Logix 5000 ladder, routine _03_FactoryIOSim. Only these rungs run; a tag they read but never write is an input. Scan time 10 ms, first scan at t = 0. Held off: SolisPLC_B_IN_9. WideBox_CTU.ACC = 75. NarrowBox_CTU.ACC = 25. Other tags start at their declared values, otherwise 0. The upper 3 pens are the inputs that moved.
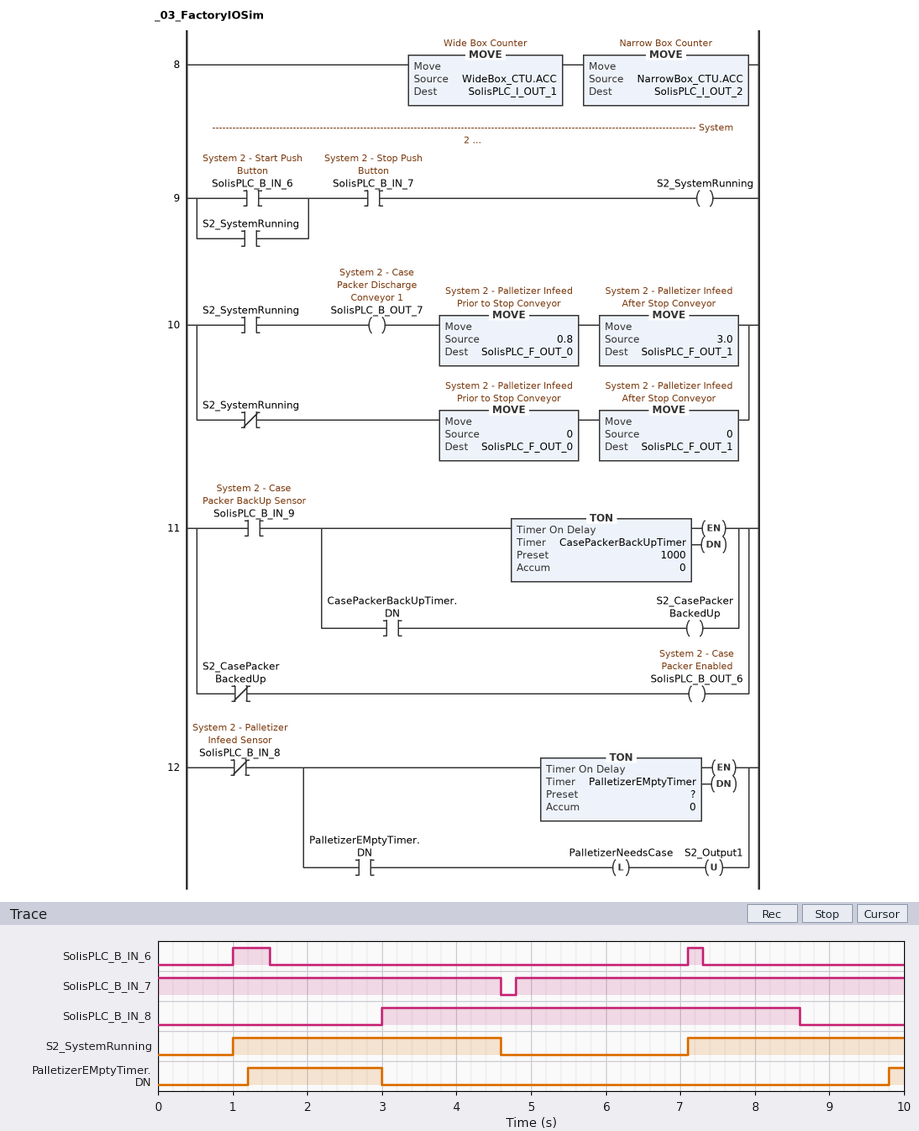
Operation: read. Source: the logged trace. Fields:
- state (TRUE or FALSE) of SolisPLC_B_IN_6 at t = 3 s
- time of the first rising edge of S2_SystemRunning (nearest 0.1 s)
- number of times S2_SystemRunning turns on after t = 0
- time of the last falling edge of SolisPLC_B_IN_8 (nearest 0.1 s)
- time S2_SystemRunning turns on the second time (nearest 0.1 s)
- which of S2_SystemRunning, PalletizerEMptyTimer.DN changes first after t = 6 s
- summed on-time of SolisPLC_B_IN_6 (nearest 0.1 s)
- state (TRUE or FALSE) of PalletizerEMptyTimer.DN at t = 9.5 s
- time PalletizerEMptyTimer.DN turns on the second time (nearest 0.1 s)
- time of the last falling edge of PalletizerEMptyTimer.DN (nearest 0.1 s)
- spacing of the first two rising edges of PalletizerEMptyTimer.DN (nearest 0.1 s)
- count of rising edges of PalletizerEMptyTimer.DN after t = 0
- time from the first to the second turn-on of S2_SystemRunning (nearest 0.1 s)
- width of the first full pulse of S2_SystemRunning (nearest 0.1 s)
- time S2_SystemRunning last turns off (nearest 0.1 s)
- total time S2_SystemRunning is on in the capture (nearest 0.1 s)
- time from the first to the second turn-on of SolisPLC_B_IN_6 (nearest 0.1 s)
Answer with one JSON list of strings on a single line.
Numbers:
["FALSE", "1.0 s", "2", "8.6 s", "7.1 s", "S2_SystemRunning", "0.7 s", "FALSE", "9.8 s", "3.0 s", "8.6 s", "2", "6.1 s", "3.6 s", "4.6 s", "6.5 s", "6.1 s"]
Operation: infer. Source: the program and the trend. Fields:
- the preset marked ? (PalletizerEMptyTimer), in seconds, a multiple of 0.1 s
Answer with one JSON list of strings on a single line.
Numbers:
["1.2 s"]
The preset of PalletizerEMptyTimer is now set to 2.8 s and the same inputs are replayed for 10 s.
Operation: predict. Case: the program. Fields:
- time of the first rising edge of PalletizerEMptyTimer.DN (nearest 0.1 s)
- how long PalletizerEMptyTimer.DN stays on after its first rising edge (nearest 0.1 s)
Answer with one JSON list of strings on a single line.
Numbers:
["2.8 s", "0.2 s"]
